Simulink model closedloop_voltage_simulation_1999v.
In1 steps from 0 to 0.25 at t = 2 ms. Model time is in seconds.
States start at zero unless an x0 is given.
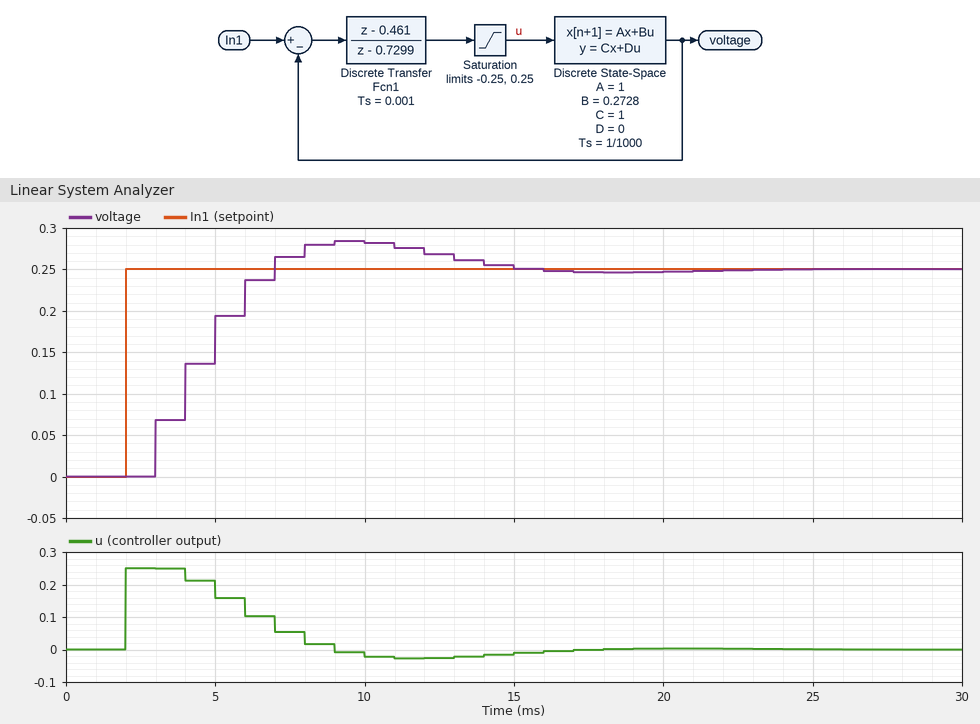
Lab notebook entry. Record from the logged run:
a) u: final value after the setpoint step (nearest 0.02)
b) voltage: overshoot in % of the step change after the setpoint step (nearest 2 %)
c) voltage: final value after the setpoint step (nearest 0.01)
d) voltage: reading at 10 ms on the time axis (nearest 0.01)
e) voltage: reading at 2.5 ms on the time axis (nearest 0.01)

0.00
14 %
0.25
0.28
0.00
